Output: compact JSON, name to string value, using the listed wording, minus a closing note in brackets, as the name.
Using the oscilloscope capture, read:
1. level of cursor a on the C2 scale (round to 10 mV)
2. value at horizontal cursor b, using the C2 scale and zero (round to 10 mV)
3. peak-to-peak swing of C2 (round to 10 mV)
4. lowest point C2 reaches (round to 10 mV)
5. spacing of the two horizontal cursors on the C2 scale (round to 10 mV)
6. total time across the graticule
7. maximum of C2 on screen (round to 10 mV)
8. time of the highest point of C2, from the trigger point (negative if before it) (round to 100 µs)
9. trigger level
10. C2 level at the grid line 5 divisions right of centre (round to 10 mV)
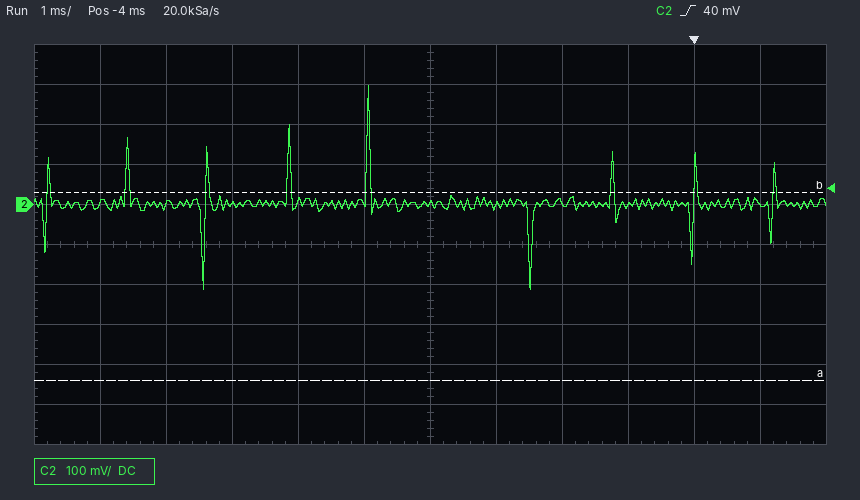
{"level of cursor a on the C2 scale": "-440 mV", "value at horizontal cursor b, using the C2 scale and zero": "30 mV", "peak-to-peak swing of C2": "510 mV", "lowest point C2 reaches": "-210 mV", "spacing of the two horizontal cursors on the C2 scale": "470 mV", "total time across the graticule": "12 ms", "maximum of C2 on screen": "300 mV", "time of the highest point of C2, from the trigger point (negative if before it)": "-4.9 ms", "trigger level": "40 mV", "C2 level at the grid line 5 divisions right of centre": "0 mV"}
